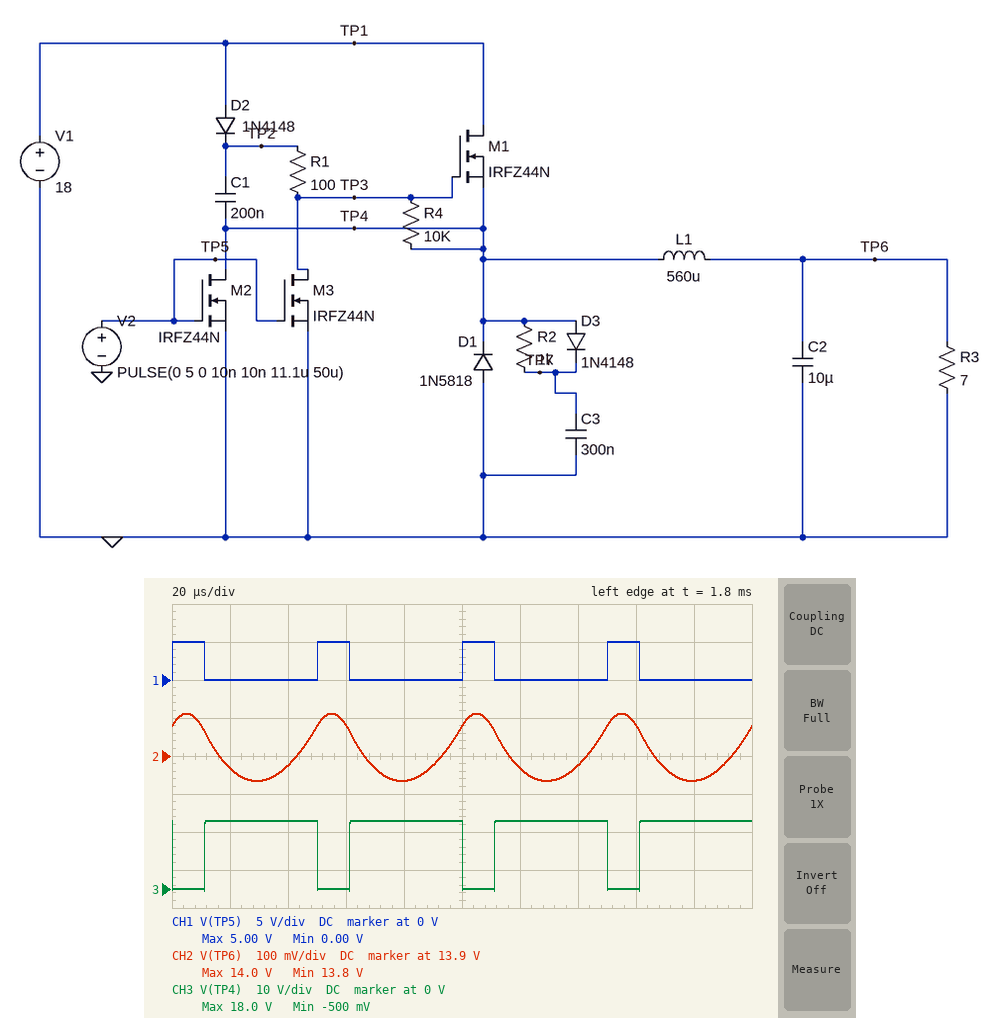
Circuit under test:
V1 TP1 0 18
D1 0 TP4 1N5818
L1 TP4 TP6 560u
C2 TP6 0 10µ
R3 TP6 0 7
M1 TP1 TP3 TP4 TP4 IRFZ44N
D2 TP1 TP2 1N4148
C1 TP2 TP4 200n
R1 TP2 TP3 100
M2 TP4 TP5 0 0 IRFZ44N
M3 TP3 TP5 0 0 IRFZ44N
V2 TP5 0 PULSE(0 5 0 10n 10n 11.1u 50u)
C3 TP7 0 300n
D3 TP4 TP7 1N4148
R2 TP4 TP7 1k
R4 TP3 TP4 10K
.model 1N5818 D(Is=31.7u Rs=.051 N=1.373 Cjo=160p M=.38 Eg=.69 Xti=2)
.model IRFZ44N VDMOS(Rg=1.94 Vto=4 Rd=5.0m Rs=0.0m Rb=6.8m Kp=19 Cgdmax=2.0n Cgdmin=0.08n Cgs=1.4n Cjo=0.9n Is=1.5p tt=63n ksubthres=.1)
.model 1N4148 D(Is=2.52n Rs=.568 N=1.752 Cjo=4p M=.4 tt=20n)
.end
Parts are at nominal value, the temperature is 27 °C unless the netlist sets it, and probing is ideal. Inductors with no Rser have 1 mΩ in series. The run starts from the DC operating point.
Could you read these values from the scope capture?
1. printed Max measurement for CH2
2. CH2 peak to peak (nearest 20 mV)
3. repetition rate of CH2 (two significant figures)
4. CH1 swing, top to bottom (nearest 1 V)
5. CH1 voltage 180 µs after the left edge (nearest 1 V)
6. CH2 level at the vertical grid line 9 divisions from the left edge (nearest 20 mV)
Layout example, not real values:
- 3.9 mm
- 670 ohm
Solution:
- 14.0 V
- 180 mV
- 20 kHz
- 5 V
- 0 V
- 13.84 V
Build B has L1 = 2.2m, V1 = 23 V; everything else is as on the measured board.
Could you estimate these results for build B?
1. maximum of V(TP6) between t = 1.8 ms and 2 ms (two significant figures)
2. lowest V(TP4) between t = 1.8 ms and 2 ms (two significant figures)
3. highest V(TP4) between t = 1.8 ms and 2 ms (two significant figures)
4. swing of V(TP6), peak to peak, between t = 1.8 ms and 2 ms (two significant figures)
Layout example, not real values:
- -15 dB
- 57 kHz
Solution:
- 18 V
- -540 mV
- 23 V
- 57 mV
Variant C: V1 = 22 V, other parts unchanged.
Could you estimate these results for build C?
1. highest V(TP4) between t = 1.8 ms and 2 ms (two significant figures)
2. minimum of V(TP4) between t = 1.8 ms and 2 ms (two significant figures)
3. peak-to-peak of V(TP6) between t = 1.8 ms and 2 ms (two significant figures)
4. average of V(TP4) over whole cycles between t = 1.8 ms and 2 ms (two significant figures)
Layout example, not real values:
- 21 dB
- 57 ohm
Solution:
- 22 V
- -520 mV
- 220 mV
- 17 V
